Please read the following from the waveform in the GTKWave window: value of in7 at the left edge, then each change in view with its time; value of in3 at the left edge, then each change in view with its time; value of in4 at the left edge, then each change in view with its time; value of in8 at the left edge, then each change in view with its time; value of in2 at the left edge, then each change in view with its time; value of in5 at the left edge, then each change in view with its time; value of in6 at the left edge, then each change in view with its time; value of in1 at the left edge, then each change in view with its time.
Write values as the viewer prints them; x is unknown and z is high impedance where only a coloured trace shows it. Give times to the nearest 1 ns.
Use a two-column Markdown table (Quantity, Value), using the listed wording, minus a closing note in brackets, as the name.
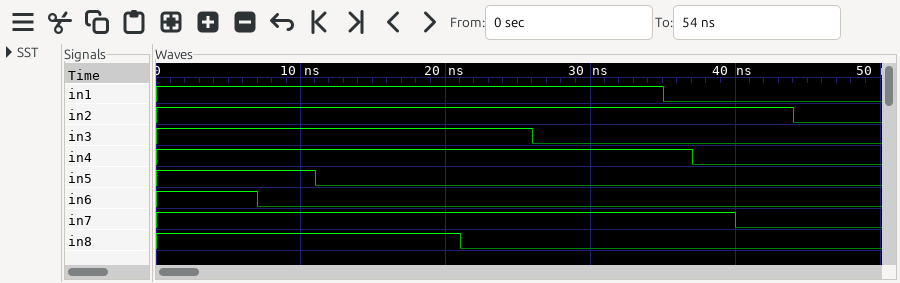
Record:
| Quantity | Value |
|---|---|
| value of in7 at the left edge, then each change in view with its time | 1, 0 at 40 ns |
| value of in3 at the left edge, then each change in view with its time | 1, 0 at 26 ns |
| value of in4 at the left edge, then each change in view with its time | 1, 0 at 37 ns |
| value of in8 at the left edge, then each change in view with its time | 1, 0 at 21 ns |
| value of in2 at the left edge, then each change in view with its time | 1, 0 at 44 ns |
| value of in5 at the left edge, then each change in view with its time | 1, 0 at 11 ns |
| value of in6 at the left edge, then each change in view with its time | 1, 0 at 7 ns |
| value of in1 at the left edge, then each change in view with its time | 1, 0 at 35 ns |
